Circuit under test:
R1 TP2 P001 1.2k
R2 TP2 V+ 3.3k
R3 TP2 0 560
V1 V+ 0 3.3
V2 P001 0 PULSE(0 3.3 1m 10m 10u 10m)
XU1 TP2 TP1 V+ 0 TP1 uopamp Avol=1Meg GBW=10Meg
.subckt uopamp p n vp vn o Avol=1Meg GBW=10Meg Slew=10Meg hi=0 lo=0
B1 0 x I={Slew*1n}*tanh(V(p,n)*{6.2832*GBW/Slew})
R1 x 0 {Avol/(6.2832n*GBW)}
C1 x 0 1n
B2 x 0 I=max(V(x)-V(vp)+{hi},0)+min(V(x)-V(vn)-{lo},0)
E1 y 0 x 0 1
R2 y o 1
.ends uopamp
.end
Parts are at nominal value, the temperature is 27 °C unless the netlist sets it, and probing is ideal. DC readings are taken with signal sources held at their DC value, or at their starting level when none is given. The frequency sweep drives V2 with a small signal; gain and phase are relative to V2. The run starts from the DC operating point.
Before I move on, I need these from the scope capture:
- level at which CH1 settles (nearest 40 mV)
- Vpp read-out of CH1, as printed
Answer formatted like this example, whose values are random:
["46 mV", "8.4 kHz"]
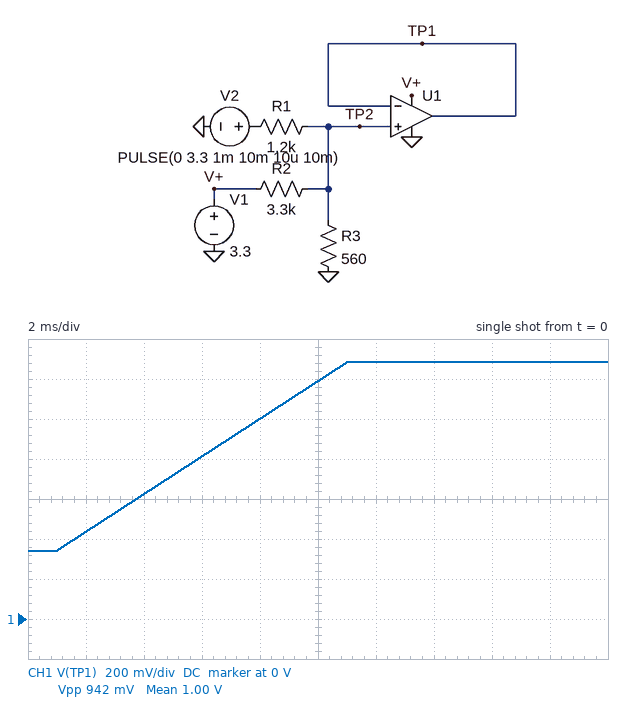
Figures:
["1.28 V", "942 mV"]
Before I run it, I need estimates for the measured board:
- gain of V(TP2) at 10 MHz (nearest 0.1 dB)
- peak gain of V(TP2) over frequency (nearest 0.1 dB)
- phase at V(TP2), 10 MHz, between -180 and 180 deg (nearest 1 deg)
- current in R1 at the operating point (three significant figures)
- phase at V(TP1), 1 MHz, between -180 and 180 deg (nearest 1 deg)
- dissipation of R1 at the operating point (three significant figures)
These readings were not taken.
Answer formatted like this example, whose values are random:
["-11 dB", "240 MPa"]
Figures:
["-10.9 dB", "-10.9 dB", "0 deg", "285 µA", "-6 deg", "97.6 µW"]
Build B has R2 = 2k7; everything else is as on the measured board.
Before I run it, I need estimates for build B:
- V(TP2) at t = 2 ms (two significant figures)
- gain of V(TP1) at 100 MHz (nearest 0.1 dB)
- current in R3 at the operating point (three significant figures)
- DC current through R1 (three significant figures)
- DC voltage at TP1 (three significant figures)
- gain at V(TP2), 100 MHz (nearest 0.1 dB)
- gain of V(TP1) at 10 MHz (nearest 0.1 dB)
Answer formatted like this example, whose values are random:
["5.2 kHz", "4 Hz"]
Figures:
["500 mV", "-31.1 dB", "730 µA", "341 µA", "409 mV", "-11.1 dB", "-14.1 dB"]
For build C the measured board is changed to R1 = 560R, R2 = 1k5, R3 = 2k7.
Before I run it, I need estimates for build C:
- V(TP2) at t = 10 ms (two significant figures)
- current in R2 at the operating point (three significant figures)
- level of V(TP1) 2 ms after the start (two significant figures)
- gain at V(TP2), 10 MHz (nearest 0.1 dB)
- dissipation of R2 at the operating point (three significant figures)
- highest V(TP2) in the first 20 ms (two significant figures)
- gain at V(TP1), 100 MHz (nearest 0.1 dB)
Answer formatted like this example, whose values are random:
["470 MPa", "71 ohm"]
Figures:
["2.7 V", "1.68 mA", "990 mV", "-4.0 dB", "4.24 mW", "2.9 V", "-24.0 dB"]
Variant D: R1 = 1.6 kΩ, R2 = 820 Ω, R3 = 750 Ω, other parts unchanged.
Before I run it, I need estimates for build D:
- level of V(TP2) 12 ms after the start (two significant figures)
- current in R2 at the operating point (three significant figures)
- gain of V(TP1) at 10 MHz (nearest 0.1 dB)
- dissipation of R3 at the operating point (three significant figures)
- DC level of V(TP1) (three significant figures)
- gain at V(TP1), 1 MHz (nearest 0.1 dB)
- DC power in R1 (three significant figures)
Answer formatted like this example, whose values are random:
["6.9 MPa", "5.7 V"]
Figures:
["1.9 V", "2.48 mA", "-17.1 dB", "2.14 mW", "1.27 V", "-14.2 dB", "1.00 mW"]
